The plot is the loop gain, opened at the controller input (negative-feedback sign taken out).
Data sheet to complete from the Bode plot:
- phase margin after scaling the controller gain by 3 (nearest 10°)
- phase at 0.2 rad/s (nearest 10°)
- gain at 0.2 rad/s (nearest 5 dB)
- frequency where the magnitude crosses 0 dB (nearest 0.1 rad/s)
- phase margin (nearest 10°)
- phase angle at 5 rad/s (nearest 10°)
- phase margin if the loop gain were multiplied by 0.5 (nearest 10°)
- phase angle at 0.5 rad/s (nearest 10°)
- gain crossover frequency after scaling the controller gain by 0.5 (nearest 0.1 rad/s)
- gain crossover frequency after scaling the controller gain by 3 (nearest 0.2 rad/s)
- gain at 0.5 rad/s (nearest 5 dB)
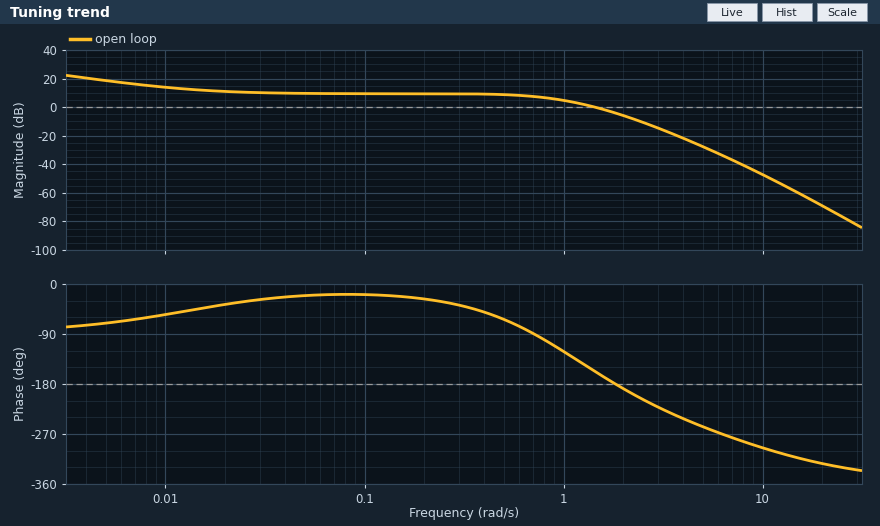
-20°
-30°
10 dB
1.4 rad/s
20°
-260°
70°
-60°
0.9 rad/s
2.4 rad/s
10 dB
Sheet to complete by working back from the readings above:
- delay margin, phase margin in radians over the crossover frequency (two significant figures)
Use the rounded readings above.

0.25 s
